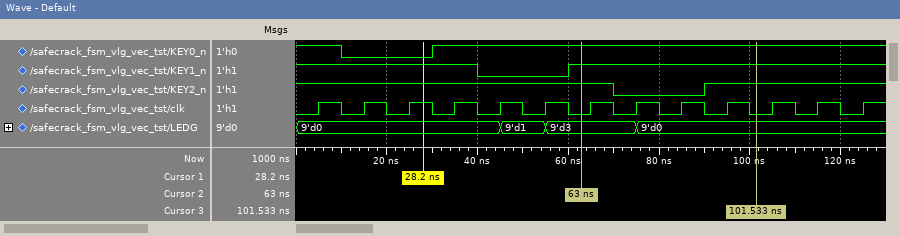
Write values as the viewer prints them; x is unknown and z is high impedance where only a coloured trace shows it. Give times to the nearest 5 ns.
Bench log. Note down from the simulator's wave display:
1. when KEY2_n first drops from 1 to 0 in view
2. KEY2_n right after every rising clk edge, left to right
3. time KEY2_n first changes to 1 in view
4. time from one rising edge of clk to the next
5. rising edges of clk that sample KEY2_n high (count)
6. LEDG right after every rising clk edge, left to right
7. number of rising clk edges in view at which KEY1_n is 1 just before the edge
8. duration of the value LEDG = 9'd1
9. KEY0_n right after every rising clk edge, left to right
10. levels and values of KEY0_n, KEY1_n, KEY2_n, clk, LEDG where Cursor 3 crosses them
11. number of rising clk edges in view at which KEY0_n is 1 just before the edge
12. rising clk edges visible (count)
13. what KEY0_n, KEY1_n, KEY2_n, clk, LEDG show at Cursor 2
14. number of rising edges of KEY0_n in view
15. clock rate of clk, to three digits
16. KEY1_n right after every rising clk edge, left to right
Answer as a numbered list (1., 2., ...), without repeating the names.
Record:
1. 70 ns
2. 1 1 1 1 1 1 1 0 0 1 1 1 1
3. 90 ns
4. 10 ns
5. 11
6. 9'd0, 9'd0, 9'd0, 9'd0, 9'd1, 9'd3, 9'd3, 9'd0, 9'd0, 9'd0, 9'd0, 9'd0, 9'd0
7. 11
8. 10 ns
9. 1 0 0 1 1 1 1 1 1 1 1 1 1
10. KEY0_n=1, KEY1_n=1, KEY2_n=1, clk=0, LEDG=9'd0
11. 11
12. 13
13. KEY0_n=1, KEY1_n=1, KEY2_n=1, clk=0, LEDG=9'd3
14. 1
15. 100 MHz
16. 1 1 1 1 0 0 1 1 1 1 1 1 1
